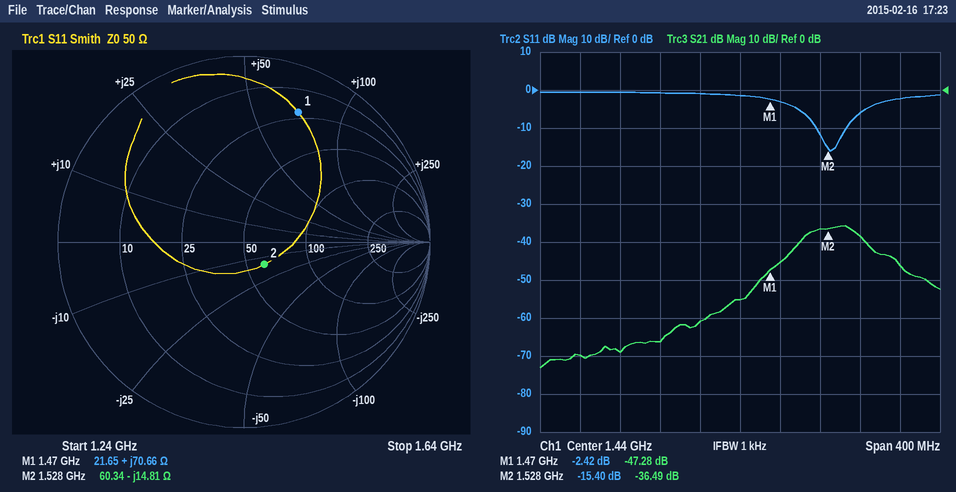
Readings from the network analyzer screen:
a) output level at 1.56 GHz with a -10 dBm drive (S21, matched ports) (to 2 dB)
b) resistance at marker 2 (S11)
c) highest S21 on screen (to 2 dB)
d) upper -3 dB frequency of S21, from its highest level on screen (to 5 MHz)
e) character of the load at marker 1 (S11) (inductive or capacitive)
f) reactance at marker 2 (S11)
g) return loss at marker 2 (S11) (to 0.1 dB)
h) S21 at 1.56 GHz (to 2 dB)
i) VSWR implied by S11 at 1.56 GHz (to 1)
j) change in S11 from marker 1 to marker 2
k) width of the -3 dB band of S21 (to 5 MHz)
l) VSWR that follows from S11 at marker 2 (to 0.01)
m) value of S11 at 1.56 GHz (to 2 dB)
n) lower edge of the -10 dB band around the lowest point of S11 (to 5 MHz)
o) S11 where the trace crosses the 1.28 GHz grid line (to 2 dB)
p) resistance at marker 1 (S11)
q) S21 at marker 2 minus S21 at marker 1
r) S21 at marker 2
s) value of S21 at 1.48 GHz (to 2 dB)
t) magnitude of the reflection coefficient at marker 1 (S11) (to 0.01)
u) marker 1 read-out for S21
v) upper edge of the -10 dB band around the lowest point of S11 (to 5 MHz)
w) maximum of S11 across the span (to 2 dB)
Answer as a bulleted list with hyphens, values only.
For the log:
- -48 dBm
- 60.34 Ω
- -36 dB
- 1.560 GHz
- inductive
- -14.81 Ω
- 15.8 dB
- -38 dB
- 3
- -12.98 dB
- 55 MHz
- 1.41
- -6 dB
- 1.515 GHz
- 0 dB
- 21.65 Ω
- 10.79 dB
- -36.49 dB
- -46 dB
- 0.76
- -47.28 dB
- 1.545 GHz
- 0 dB
